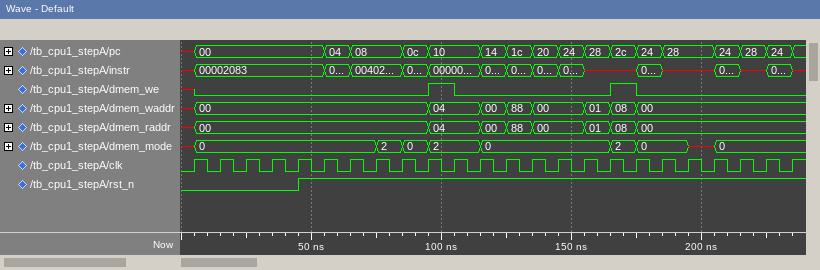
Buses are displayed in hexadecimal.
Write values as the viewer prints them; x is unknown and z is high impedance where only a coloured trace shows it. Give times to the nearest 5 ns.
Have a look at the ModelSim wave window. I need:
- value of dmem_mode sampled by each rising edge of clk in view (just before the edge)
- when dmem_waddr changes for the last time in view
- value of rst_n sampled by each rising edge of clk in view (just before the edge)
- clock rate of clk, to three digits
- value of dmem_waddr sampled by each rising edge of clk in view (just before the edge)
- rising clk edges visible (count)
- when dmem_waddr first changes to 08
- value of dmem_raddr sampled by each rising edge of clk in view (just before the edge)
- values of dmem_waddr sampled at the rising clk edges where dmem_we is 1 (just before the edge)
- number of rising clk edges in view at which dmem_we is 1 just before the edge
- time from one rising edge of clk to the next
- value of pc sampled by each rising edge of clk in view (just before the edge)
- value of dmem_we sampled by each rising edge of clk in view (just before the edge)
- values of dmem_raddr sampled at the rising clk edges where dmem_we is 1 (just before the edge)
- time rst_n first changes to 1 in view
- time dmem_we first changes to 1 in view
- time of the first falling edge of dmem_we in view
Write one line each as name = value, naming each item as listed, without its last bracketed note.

value of dmem_mode sampled by each rising edge of clk in view = x, 0, 0, 0, 0, 0, 0, 0, 2, 0, 2, 2, 0, 0, 0, 0, 0, 2, 0, 0, x, 0, 0, 0
when dmem_waddr changes for the last time in view = 175 ns
value of rst_n sampled by each rising edge of clk in view = 0 0 0 0 0 1 1 1 1 1 1 1 1 1 1 1 1 1 1 1 1 1 1 1
clock rate of clk, to three digits = 100 MHz
value of dmem_waddr sampled by each rising edge of clk in view = x, 00, 00, 00, 00, 00, 00, 00, 00, 00, 04, 04, 00, 88, 00, 00, 01, 08, 00, 00, 00, 00, 00, 00
rising clk edges visible = 24
when dmem_waddr first changes to 08 = 165 ns
value of dmem_raddr sampled by each rising edge of clk in view = x, 00, 00, 00, 00, 00, 00, 00, 00, 00, 04, 04, 00, 88, 00, 00, 01, 08, 00, 00, 00, 00, 00, 00
values of dmem_waddr sampled at the rising clk edges where dmem_we is 1 = 04, 08
number of rising clk edges in view at which dmem_we is 1 just before the edge = 2
time from one rising edge of clk to the next = 10 ns
value of pc sampled by each rising edge of clk in view = x, 00, 00, 00, 00, 00, 04, 08, 08, 0c, 10, 10, 14, 1c, 20, 24, 28, 2c, 24, 28, 28, 24, 28, 24
value of dmem_we sampled by each rising edge of clk in view = x 0 0 0 0 0 0 0 0 0 1 0 0 0 0 0 0 1 0 0 0 0 0 0
values of dmem_raddr sampled at the rising clk edges where dmem_we is 1 = 04, 08
time rst_n first changes to 1 in view = 45 ns
time dmem_we first changes to 1 in view = 95 ns
time of the first falling edge of dmem_we in view = 105 ns
